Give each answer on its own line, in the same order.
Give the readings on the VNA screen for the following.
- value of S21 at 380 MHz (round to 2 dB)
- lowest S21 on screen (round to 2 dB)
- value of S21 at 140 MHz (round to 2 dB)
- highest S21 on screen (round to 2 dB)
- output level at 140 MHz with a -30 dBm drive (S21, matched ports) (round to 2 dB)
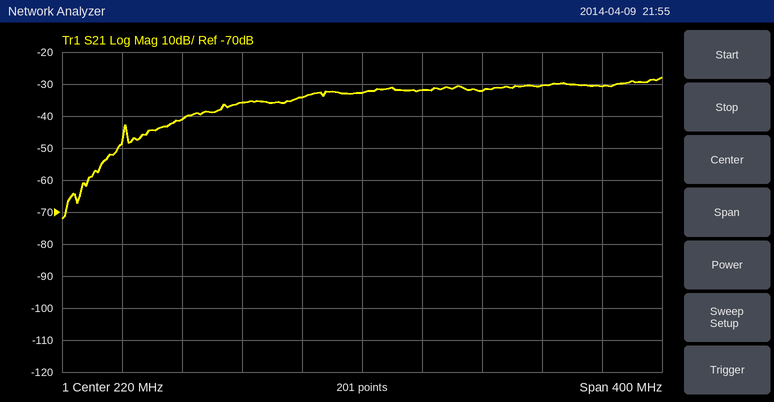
-30 dB
-72 dB
-36 dB
-28 dB
-66 dBm
